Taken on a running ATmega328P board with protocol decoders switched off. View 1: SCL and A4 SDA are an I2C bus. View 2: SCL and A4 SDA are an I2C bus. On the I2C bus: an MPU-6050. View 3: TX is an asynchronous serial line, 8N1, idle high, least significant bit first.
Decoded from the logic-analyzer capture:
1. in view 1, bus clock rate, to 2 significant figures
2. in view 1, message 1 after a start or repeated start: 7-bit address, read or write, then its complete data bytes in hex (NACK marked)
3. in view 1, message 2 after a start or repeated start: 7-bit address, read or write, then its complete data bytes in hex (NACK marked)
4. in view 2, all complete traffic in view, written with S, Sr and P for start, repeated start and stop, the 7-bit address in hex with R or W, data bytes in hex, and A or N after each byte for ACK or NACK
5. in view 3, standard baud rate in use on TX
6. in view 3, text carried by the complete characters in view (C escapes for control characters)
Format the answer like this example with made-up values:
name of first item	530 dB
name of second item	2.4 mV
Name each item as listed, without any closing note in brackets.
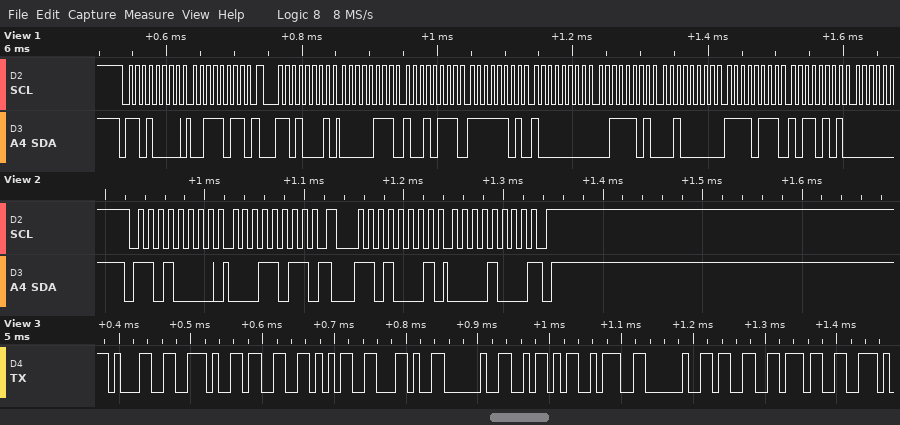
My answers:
in view 1, bus clock rate, to 2 significant figures	100 kHz
in view 1, message 1 after a start or repeated start: 7-bit address, read or write, then its complete data bytes in hex	0x68 write: 3B
in view 1, message 2 after a start or repeated start: 7-bit address, read or write, then its complete data bytes in hex	0x68 read: 07 97 FD 80 3D 20 F7 B5
in view 2, all complete traffic in view, written with S, Sr and P for start, repeated start and stop, the 7-bit address in hex with R or W, data bytes in hex, and A or N after each byte for ACK or NACK	S 68W A 1B A Sr 68R A 08 N P
in view 3, standard baud rate in use on TX	115200 baud
in view 3, text carried by the complete characters in view	"1.35, Z: 37"
